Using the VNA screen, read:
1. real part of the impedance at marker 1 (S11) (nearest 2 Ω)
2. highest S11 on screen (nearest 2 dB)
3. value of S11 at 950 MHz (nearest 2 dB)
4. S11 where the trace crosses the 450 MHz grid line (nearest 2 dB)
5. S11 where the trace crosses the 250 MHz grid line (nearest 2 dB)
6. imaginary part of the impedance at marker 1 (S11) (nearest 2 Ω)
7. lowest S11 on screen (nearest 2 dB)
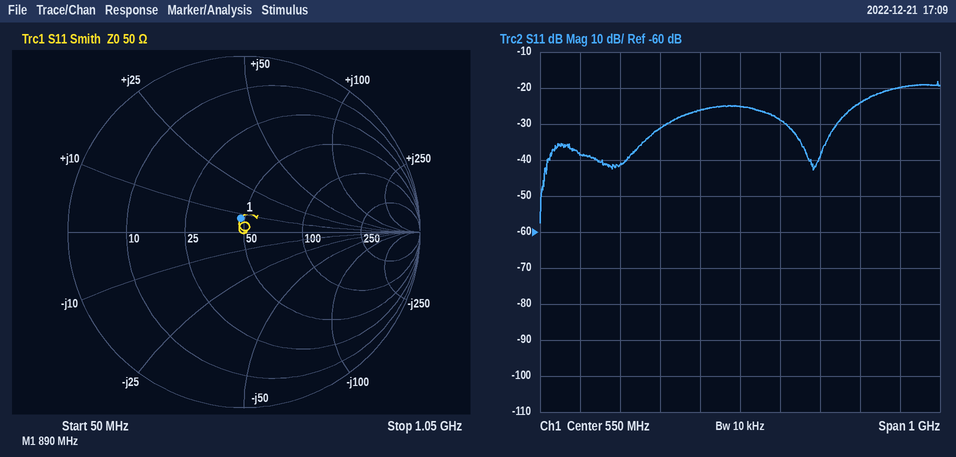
48 Ω
-18 dB
-20 dB
-26 dB
-42 dB
+8 Ω
-58 dB
